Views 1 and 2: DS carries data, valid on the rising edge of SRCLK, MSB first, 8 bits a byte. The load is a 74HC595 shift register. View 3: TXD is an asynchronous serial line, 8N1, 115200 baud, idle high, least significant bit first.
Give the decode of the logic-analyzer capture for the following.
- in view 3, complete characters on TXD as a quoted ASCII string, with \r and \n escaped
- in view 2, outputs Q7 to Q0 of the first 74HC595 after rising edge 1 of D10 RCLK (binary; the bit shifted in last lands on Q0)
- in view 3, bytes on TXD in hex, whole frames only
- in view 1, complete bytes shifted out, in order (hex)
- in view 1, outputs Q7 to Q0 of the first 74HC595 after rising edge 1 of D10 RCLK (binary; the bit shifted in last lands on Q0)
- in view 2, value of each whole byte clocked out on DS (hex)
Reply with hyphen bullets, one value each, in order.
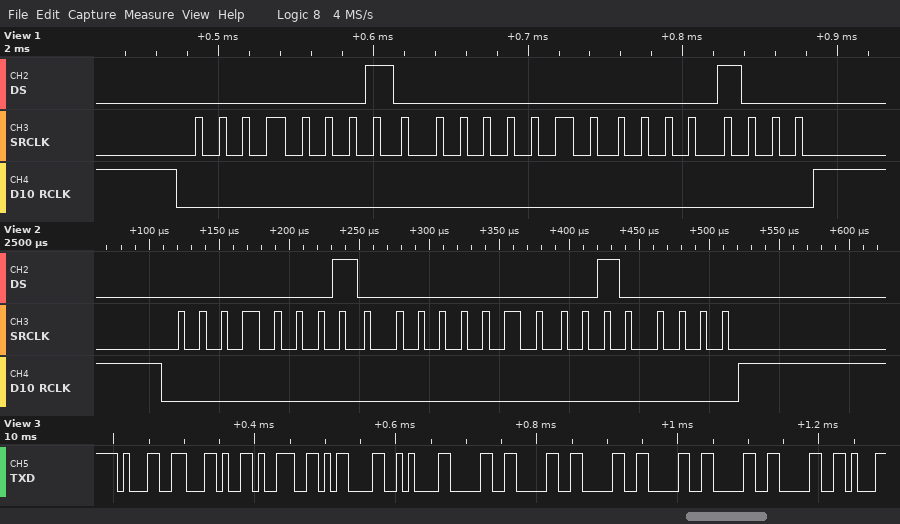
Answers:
- "1,9\r\n000000"
- 00100000
- 31 2C 39 0D 0A 30 30 30 30 30 30
- 0x01 0x00 0x08
- 00001000
- 0x01 0x00 0x20
